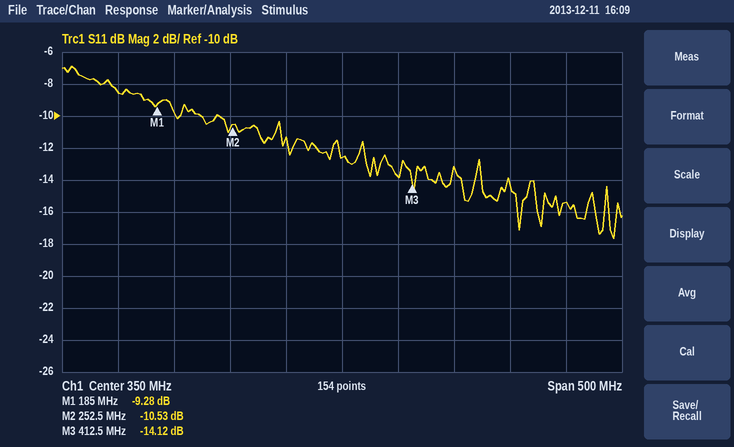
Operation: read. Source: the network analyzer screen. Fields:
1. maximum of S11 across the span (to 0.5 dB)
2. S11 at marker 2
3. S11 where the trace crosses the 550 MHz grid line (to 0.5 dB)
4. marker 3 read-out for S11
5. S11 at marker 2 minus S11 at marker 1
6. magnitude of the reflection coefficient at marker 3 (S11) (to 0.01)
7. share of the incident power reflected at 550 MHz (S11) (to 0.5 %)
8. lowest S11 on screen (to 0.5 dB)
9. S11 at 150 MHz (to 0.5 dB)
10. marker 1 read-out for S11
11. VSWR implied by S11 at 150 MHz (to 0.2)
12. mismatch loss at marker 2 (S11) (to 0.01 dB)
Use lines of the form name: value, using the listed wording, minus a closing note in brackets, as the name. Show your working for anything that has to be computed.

maximum of S11 across the span: -7.0 dB
S11 at marker 2: -10.53 dB
S11 where the trace crosses the 550 MHz grid line: -15.5 dB
marker 3 read-out for S11: -14.12 dB
S11 at marker 2 minus S11 at marker 1: -10.53 − (-9.28) = -1.25 dB
magnitude of the reflection coefficient at marker 3 (S11): 10^(-14.12/20) ≈ 0.20
share of the incident power reflected at 550 MHz (S11): 10^(-15.5/10) ≈ 2.82 %, so 3.0 % to the nearest 0.5 %
lowest S11 on screen: -17.5 dB
S11 at 150 MHz: -8.5 dB
marker 1 read-out for S11: -9.28 dB
VSWR implied by S11 at 150 MHz: |Γ| = 10^(-8.5/20) = 0.3758; VSWR = (1 + 0.3758)/(1 − 0.3758) ≈ 2.2
mismatch loss at marker 2 (S11): −10 log10(1 − 10^(-10.53/10)) ≈ 0.40 dB
